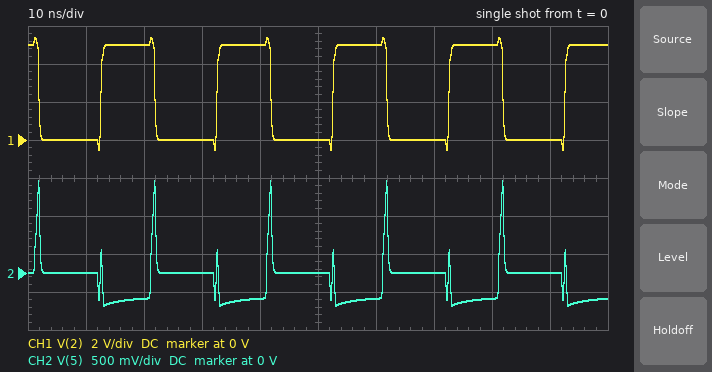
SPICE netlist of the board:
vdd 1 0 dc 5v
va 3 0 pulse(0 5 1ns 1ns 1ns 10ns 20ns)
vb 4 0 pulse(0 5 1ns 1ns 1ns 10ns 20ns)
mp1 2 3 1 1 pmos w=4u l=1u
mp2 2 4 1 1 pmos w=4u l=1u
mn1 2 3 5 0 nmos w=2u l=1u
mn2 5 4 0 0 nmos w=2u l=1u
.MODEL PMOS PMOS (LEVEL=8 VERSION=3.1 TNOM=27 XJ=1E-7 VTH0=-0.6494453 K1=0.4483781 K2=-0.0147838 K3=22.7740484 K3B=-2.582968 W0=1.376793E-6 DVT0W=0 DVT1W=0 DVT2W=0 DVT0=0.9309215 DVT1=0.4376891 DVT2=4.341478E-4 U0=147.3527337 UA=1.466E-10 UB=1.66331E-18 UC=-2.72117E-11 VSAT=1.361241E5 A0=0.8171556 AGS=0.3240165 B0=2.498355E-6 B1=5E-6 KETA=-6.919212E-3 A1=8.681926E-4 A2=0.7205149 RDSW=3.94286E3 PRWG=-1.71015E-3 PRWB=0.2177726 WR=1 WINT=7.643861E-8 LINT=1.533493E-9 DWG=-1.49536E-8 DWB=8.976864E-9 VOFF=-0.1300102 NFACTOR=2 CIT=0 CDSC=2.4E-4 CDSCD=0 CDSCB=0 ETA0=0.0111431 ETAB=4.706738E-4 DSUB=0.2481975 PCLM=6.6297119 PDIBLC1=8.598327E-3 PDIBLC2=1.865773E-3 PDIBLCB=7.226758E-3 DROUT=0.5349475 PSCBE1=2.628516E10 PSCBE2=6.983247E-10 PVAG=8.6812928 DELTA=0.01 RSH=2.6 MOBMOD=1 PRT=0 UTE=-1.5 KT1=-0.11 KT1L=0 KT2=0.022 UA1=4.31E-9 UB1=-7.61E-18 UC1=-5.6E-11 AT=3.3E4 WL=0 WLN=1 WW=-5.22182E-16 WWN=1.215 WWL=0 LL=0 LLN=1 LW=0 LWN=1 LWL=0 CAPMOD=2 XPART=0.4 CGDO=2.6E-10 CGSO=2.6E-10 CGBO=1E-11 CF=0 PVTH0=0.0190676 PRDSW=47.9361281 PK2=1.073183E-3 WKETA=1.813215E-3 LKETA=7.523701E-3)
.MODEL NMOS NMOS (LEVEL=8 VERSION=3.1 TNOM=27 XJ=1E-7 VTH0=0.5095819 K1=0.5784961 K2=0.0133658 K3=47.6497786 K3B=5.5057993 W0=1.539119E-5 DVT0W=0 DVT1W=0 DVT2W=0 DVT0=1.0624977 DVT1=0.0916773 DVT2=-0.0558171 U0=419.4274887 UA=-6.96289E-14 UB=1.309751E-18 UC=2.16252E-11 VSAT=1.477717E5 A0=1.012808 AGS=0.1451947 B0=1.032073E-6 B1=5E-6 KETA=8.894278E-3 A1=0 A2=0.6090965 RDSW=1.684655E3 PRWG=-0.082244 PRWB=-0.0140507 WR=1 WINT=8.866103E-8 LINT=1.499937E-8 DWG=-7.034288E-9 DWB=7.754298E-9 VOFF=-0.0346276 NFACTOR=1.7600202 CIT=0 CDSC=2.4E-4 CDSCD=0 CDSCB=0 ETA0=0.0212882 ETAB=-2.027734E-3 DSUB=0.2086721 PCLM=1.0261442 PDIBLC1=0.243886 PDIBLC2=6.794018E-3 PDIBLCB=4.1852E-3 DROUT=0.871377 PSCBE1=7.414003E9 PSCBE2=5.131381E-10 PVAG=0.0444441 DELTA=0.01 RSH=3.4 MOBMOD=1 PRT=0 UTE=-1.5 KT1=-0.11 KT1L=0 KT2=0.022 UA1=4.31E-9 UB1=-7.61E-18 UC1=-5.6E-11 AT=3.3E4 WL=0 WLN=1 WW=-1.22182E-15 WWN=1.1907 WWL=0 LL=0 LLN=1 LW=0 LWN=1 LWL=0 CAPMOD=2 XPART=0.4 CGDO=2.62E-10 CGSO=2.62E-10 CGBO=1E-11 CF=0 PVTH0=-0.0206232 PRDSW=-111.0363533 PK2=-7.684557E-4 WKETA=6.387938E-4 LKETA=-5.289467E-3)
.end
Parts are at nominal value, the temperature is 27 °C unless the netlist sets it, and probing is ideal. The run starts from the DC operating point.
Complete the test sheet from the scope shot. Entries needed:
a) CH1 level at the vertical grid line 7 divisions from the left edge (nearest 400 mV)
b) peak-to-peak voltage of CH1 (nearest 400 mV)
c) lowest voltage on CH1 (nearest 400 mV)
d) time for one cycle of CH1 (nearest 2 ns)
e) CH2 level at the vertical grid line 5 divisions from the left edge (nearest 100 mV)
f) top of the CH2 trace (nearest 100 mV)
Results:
0 V
6.0 V
-400 mV
20 ns
0 V
1.2 V
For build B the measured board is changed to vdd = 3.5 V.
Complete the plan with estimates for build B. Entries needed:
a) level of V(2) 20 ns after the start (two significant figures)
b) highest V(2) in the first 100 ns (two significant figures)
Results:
3.5 V
3.9 V
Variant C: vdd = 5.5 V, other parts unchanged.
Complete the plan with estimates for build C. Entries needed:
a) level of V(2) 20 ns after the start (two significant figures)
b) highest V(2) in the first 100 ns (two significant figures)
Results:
5.5 V
5.9 V
